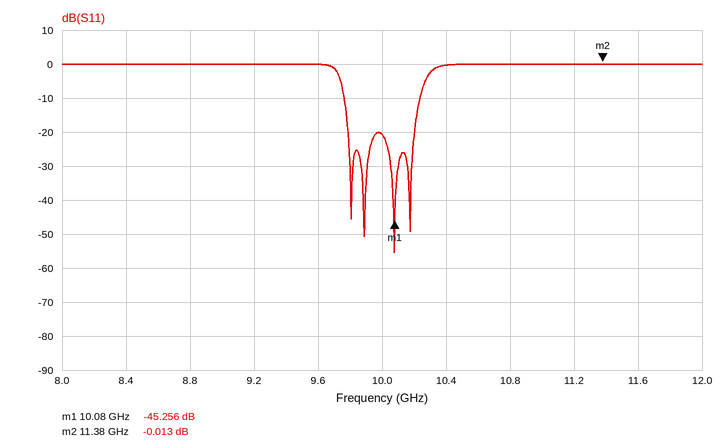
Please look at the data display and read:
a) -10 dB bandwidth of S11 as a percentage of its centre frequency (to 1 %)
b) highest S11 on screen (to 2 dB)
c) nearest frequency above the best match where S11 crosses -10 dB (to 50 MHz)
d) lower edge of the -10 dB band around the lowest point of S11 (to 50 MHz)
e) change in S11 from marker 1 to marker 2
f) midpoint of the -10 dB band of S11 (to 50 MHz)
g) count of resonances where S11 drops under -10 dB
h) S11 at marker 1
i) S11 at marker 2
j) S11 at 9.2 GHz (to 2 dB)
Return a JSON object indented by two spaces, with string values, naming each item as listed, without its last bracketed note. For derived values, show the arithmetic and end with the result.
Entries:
{
  "-10 dB bandwidth of S11 as a percentage of its centre frequency": "500 MHz / 10 GHz ≈ 5 %",
  "highest S11 on screen": "0 dB",
  "nearest frequency above the best match where S11 crosses -10 dB": "10.25 GHz",
  "lower edge of the -10 dB band around the lowest point of S11": "9.75 GHz",
  "change in S11 from marker 1 to marker 2": "-0.013 − (-45.256) = 45.243 dB",
  "midpoint of the -10 dB band of S11": "10.00 GHz",
  "count of resonances where S11 drops under -10 dB": "4",
  "S11 at marker 1": "-45.256 dB",
  "S11 at marker 2": "-0.013 dB",
  "S11 at 9.2 GHz": "0 dB"
}
